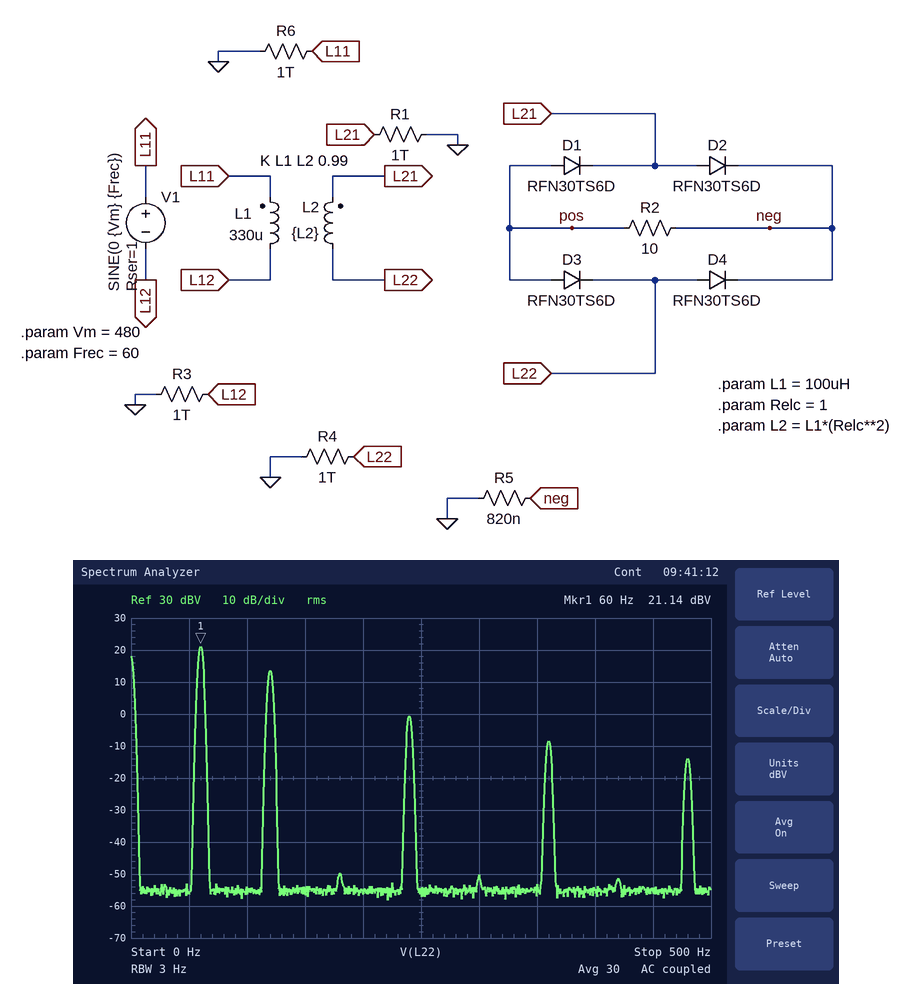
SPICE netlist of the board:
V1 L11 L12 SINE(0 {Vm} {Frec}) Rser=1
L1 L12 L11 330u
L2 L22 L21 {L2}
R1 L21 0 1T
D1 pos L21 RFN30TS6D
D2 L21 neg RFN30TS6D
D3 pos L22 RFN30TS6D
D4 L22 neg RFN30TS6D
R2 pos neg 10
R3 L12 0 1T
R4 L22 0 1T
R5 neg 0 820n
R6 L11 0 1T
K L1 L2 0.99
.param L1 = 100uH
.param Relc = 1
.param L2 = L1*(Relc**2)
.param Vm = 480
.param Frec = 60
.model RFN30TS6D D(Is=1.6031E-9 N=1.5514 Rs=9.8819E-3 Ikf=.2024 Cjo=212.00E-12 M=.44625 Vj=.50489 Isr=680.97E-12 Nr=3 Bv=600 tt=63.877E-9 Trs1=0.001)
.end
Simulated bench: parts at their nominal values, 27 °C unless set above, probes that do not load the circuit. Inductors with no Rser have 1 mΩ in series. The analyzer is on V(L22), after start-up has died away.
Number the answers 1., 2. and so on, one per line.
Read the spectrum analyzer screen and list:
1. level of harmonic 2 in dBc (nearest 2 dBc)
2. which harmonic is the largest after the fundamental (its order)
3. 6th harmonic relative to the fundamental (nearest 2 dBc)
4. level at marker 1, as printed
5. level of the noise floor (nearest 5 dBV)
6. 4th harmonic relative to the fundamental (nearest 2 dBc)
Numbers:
1. -8 dBc
2. 2
3. -30 dBc
4. 21.14 dBV
5. -55 dBV
6. -22 dBc
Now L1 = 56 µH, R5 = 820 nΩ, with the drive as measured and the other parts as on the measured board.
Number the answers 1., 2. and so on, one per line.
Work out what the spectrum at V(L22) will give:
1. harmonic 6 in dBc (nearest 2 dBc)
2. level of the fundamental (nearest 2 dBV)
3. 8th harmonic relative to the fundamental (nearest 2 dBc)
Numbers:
1. -32 dBc
2. 14 dBV
3. -38 dBc
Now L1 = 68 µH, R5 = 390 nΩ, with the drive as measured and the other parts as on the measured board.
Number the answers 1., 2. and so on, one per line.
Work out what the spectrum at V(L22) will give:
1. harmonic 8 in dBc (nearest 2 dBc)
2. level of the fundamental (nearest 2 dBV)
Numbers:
1. -38 dBc
2. 14 dBV
